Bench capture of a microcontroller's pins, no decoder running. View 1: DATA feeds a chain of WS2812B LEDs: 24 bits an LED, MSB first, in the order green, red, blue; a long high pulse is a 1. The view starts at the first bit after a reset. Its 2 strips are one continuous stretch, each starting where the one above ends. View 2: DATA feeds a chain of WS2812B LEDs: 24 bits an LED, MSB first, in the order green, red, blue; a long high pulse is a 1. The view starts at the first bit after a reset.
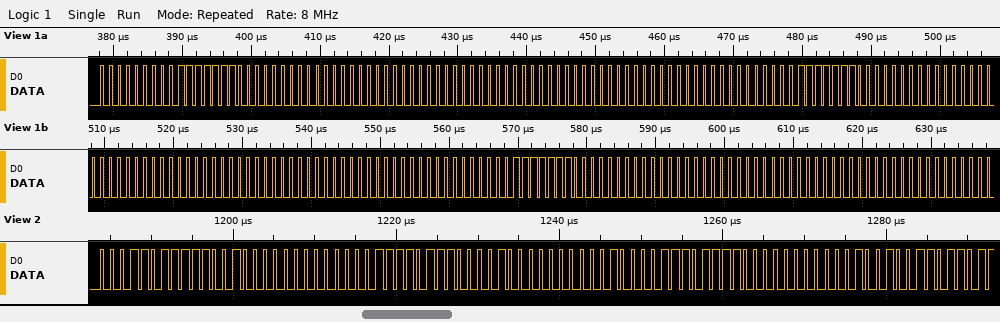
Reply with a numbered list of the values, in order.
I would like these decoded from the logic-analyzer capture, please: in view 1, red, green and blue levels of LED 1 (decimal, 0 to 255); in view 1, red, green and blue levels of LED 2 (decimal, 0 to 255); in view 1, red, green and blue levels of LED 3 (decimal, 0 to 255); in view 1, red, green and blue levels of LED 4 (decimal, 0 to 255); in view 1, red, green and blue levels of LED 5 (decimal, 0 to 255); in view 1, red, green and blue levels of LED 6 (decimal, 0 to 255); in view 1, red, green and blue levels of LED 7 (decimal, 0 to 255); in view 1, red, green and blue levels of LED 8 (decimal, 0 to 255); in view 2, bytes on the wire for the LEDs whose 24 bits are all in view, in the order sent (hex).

1. 127, 0, 0
2. 0, 0, 0
3. 0, 0, 0
4. 127, 0, 0
5. 0, 0, 0
6. 0, 0, 0
7. 127, 0, 0
8. 0, 0, 0
9. 1B E4 00 1E E1 00 21 DE 00
